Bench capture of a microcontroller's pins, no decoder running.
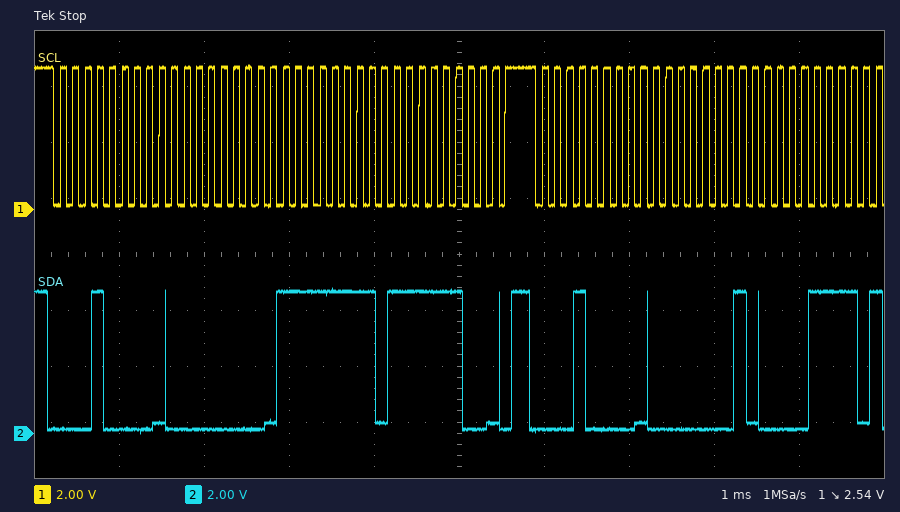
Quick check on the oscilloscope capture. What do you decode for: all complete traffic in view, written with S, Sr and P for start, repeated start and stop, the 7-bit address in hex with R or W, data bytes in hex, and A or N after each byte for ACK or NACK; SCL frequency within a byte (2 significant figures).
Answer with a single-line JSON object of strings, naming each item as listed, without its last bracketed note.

{"all complete traffic in view, written with S, Sr and P for start, repeated start and stop, the 7-bit address in hex with R or W, data bytes in hex, and A or N after each byte for ACK or NACK": "S 08W A 00 A FF A FC A P S 08W A 01 A 0F A", "SCL frequency within a byte": "6.9 kHz"}
